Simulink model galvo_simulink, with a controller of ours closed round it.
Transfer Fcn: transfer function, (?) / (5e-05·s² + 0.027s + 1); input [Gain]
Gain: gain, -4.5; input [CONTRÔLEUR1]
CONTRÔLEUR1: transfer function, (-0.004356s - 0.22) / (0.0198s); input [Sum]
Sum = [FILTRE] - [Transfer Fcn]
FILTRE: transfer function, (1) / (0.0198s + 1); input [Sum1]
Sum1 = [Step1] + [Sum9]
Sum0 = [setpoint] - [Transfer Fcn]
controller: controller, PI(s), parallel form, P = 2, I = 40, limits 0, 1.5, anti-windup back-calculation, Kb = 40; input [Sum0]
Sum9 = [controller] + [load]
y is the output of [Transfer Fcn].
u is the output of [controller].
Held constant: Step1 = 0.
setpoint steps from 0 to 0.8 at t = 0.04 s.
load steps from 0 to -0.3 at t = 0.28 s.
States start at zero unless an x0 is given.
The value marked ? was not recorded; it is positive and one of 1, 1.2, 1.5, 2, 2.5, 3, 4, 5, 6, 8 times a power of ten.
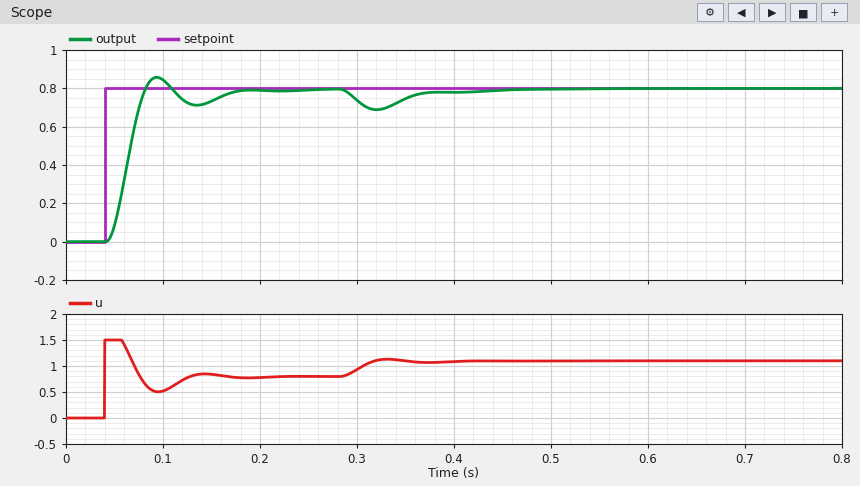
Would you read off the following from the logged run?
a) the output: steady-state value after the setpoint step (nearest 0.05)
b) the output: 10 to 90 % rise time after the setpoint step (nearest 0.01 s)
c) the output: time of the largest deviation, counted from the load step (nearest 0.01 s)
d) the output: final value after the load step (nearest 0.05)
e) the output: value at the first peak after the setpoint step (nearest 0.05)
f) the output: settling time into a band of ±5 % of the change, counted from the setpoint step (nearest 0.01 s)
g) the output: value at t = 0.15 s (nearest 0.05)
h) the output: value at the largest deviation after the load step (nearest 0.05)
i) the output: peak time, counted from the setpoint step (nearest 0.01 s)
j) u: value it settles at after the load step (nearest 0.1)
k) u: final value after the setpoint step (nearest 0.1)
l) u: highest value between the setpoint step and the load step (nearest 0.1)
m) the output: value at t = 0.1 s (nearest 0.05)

0.80
0.03 s
0.04 s
0.80
0.85
0.12 s
0.75
0.70
0.05 s
1.1
0.8
1.5
0.85
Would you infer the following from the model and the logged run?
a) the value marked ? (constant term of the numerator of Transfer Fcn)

1
